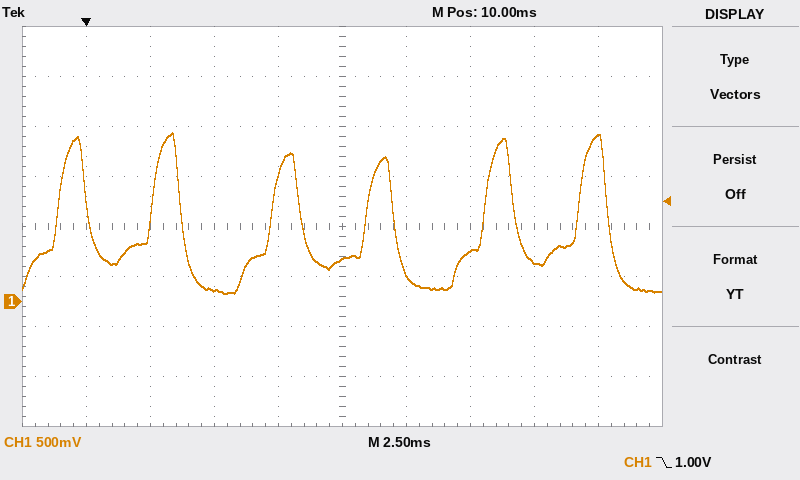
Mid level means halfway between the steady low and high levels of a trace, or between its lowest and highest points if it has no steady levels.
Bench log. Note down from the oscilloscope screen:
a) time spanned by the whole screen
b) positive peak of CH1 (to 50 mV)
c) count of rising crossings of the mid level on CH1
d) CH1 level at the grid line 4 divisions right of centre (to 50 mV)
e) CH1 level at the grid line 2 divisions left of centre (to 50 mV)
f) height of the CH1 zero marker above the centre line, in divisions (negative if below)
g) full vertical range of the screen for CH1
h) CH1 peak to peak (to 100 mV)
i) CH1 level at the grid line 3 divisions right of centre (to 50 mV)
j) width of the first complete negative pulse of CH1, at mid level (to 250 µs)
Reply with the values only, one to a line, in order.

25 ms
1.70 V
6
1.65 V
100 mV
-1.5 div
4 V
1.60 V
400 mV
2.50 ms
